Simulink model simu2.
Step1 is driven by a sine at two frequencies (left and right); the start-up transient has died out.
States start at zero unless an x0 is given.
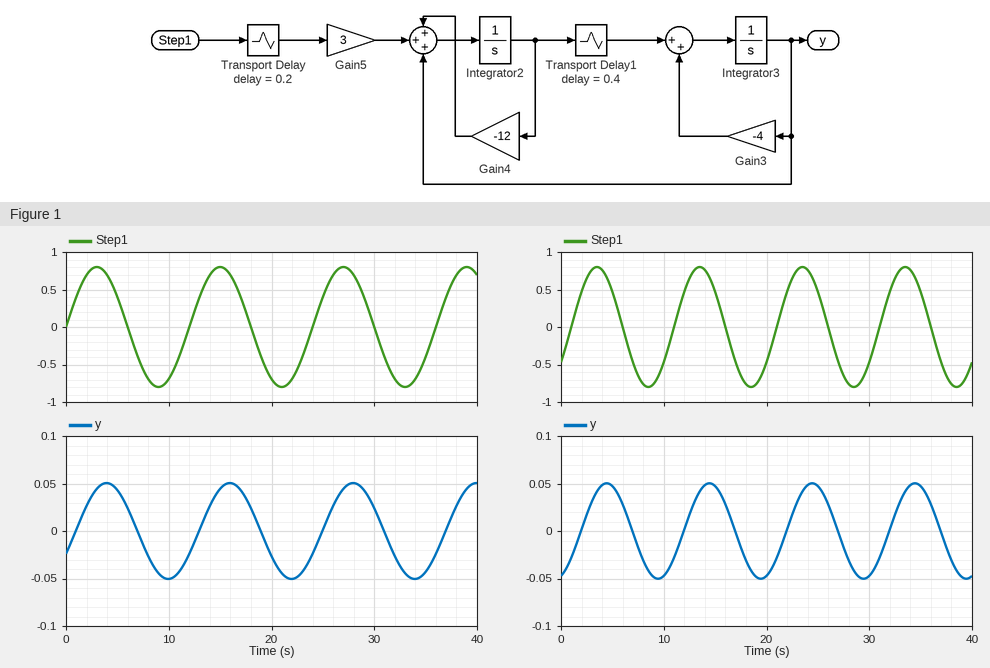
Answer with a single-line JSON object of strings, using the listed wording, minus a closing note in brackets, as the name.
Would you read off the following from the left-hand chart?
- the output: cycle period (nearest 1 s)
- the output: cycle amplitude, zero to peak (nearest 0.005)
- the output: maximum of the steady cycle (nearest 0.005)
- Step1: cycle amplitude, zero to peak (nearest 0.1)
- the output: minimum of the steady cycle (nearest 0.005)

{"the output: cycle period": "12 s", "the output: cycle amplitude, zero to peak": "0.050", "the output: maximum of the steady cycle": "0.050", "Step1: cycle amplitude, zero to peak": "0.8", "the output: minimum of the steady cycle": "-0.050"}
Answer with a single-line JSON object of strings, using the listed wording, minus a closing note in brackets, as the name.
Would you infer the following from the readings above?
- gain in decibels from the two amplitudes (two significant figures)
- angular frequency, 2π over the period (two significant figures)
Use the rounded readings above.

{"gain in decibels from the two amplitudes": "-24 dB", "angular frequency, 2π over the period": "0.52 rad/s"}
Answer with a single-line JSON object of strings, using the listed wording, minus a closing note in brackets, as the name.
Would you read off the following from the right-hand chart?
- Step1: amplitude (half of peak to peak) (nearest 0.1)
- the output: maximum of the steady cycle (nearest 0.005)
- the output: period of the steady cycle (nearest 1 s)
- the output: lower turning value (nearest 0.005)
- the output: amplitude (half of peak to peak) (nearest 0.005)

{"Step1: amplitude (half of peak to peak)": "0.8", "the output: maximum of the steady cycle": "0.050", "the output: period of the steady cycle": "10 s", "the output: lower turning value": "-0.050", "the output: amplitude (half of peak to peak)": "0.050"}
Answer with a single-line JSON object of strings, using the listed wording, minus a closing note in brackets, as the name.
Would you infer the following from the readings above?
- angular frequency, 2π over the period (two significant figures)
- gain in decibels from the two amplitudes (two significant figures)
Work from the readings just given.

{"angular frequency, 2π over the period": "0.63 rad/s", "gain in decibels from the two amplitudes": "-24 dB"}
